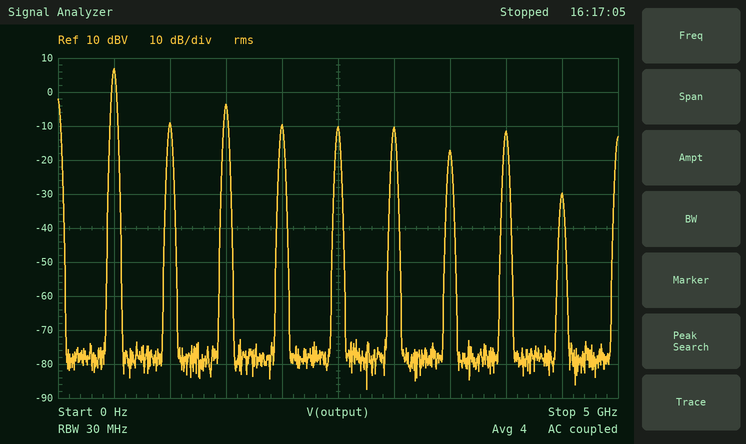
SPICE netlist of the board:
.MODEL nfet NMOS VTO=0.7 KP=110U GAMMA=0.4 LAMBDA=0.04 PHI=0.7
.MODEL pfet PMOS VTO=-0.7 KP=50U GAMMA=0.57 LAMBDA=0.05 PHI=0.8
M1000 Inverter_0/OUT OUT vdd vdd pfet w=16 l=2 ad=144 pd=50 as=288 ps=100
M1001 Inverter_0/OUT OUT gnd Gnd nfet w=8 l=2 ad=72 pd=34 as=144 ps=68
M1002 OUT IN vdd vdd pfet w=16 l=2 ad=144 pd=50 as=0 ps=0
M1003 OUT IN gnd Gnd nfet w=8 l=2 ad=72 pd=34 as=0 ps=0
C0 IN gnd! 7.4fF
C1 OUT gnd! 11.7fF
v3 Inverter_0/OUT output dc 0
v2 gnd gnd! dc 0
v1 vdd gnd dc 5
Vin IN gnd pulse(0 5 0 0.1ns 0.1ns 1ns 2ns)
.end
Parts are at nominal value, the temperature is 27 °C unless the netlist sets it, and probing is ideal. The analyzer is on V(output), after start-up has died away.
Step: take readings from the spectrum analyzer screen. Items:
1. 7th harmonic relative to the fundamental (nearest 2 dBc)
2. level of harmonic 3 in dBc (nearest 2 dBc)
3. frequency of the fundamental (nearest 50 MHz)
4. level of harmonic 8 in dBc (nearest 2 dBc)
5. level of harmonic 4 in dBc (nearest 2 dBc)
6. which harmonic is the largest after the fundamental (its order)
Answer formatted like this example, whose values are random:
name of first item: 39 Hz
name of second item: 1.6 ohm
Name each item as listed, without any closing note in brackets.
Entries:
7th harmonic relative to the fundamental: -24 dBc
level of harmonic 3 in dBc: -10 dBc
frequency of the fundamental: 500 MHz
level of harmonic 8 in dBc: -18 dBc
level of harmonic 4 in dBc: -16 dBc
which harmonic is the largest after the fundamental: 3
